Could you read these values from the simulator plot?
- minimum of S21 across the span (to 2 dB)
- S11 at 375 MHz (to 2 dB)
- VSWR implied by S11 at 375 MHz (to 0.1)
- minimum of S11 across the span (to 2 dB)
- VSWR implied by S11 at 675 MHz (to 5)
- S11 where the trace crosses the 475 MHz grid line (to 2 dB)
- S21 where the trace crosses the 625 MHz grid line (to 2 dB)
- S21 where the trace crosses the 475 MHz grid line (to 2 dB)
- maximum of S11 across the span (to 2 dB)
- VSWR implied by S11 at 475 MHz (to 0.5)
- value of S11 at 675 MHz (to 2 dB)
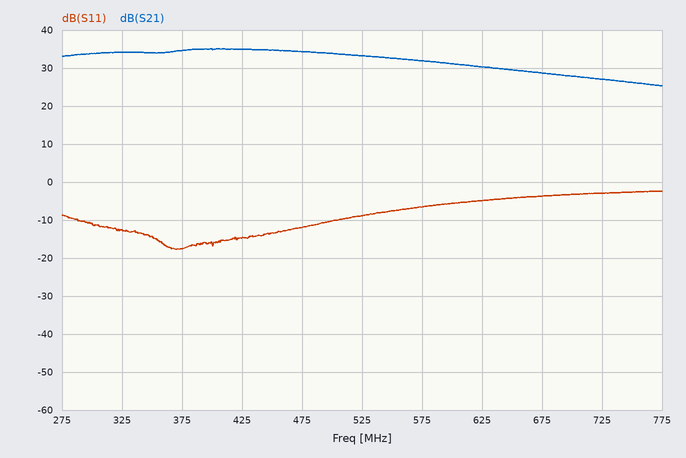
26 dB
-18 dB
1.3
-18 dB
5
-12 dB
30 dB
34 dB
-2 dB
1.5
-4 dB
